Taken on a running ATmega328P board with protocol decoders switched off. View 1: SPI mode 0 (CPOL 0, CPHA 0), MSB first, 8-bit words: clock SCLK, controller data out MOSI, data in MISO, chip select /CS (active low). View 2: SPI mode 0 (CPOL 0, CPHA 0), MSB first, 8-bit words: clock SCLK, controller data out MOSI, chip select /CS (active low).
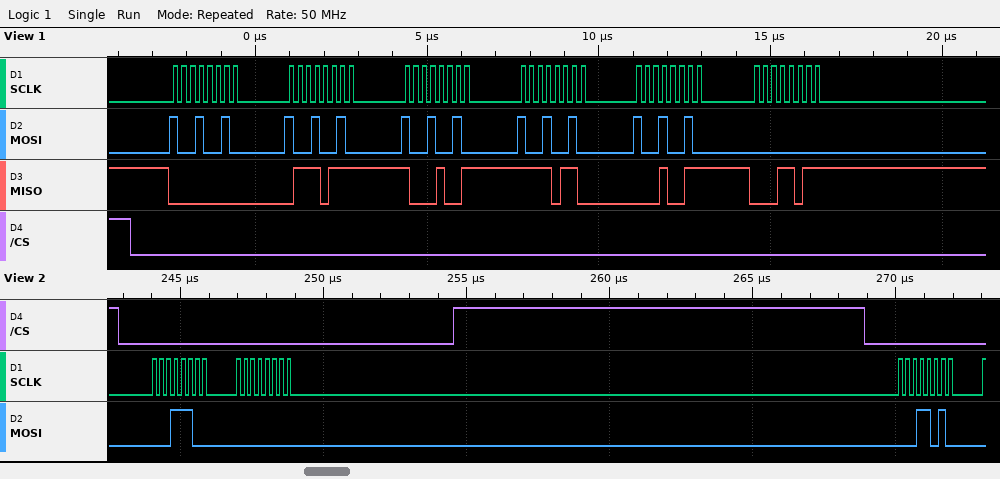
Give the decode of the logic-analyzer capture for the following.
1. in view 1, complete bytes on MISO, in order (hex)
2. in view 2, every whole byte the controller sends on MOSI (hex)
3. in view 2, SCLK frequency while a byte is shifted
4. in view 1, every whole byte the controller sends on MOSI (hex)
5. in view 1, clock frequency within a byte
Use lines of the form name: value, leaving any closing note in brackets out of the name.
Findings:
in view 1, complete bytes on MISO, in order: 0x00 0x77 0x89 0xF6 0x13 0x1B
in view 2, every whole byte the controller sends on MOSI: 1C 00 1A
in view 2, SCLK frequency while a byte is shifted: 4 MHz
in view 1, every whole byte the controller sends on MOSI: 0x92 0x92 0x92 0x92 0x92 0x00
in view 1, clock frequency within a byte: 4 MHz
